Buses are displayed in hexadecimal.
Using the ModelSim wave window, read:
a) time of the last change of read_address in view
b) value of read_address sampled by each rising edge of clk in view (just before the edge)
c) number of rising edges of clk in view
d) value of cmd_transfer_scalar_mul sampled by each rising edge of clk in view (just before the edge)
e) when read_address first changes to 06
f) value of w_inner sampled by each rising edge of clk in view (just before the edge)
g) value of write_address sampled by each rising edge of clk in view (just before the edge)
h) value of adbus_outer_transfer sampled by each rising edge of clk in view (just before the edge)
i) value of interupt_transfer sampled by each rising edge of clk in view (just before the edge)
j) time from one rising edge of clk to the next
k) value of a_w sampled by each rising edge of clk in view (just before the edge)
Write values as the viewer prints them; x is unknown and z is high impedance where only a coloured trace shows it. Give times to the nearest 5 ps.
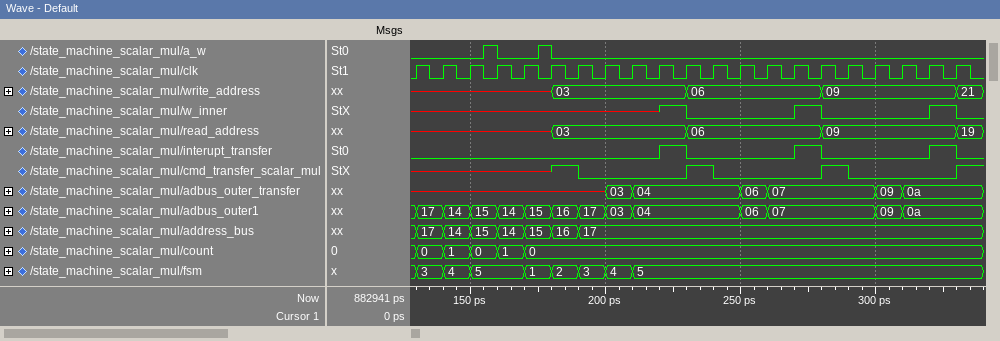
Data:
330 ps
x, x, x, x, x, x, 03, 03, 03, 03, 03, 06, 06, 06, 06, 06, 09, 09, 09, 09, 09
21
x x x x x x 1 0 0 0 0 1 0 0 0 0 1 0 0 0 0
230 ps
x x x x x x x x x x 1 0 0 0 0 1 0 0 0 0 1
x, x, x, x, x, x, 03, 03, 03, 03, 03, 06, 06, 06, 06, 06, 09, 09, 09, 09, 09
x, x, x, x, x, x, x, x, 03, 04, 04, 04, 04, 06, 07, 07, 07, 07, 09, 0a, 0a
0 0 0 0 0 0 0 0 0 0 1 0 0 0 0 1 0 0 0 0 1
10 ps
0 0 0 1 0 1 0 0 0 0 0 0 0 0 0 0 0 0 0 0 0
